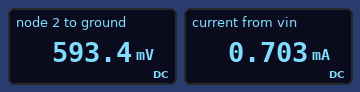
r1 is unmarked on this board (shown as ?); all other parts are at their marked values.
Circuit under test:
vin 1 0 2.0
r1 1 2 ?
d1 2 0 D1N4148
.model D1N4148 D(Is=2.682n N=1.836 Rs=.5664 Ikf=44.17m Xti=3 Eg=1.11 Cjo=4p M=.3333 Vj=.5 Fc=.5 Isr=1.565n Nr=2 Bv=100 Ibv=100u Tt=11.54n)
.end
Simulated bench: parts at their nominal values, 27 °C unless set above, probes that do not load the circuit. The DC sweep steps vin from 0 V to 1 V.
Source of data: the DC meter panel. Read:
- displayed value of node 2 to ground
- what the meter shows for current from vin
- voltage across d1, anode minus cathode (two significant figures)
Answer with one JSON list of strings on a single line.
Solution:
["593.4 mV", "0.703 mA", "590 mV"]
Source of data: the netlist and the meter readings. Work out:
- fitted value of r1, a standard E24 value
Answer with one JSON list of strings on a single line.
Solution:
["2 kΩ"]
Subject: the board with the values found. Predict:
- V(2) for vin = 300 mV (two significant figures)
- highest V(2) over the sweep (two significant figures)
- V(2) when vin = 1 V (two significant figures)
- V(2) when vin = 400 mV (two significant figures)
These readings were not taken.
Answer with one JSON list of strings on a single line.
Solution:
["300 mV", "540 mV", "540 mV", "380 mV"]
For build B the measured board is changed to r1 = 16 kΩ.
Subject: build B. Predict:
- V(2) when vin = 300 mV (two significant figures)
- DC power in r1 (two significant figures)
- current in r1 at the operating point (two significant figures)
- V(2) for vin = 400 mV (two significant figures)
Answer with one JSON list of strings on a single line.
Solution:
["280 mV", "140 µW", "94 µA", "340 mV"]
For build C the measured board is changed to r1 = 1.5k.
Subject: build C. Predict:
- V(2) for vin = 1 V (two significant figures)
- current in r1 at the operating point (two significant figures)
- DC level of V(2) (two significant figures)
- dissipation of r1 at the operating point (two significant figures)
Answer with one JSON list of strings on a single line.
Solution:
["550 mV", "930 µA", "610 mV", "1.3 mW"]
